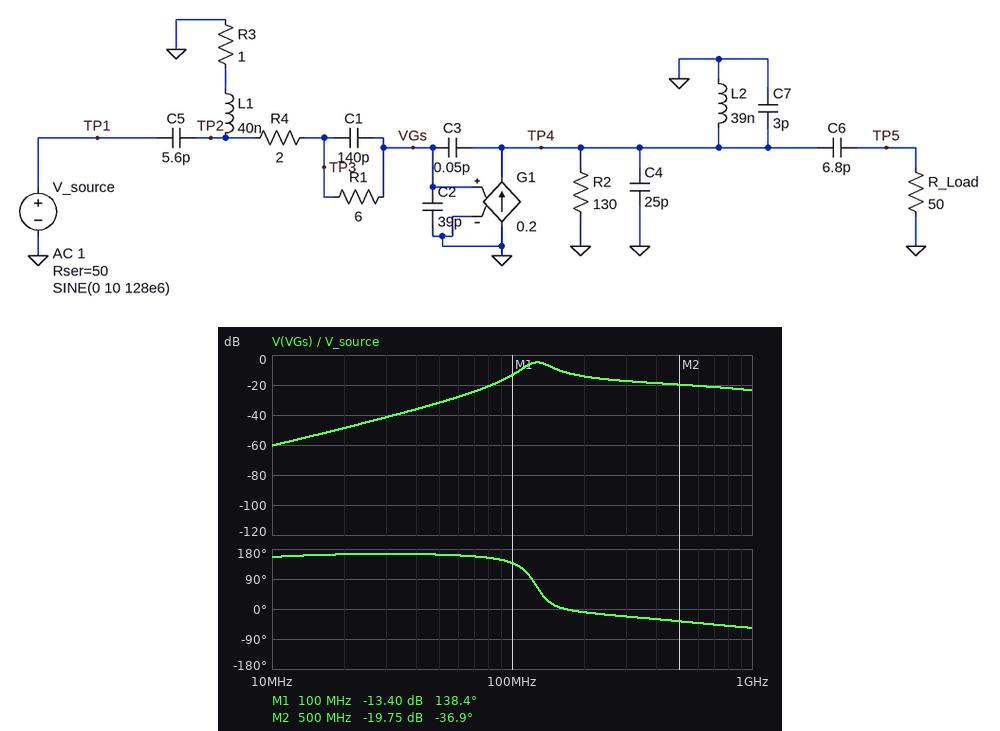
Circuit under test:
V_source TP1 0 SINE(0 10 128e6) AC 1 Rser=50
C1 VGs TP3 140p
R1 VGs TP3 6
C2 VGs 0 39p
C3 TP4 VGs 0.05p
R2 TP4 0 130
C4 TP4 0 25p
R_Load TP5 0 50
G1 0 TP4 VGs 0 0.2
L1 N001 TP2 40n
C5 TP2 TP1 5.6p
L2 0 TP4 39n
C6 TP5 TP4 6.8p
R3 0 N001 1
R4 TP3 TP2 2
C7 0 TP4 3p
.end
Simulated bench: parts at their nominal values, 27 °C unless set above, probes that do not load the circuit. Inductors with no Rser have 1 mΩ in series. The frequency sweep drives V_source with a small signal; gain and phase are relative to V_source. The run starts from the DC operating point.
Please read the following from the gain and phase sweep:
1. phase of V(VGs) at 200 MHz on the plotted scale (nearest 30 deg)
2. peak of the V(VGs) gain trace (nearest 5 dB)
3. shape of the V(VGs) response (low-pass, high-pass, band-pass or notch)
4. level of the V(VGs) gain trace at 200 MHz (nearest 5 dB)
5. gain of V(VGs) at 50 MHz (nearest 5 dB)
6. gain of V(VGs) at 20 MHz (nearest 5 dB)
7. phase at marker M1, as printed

0 deg
-5 dB
band-pass
-15 dB
-30 dB
-50 dB
138.4 deg
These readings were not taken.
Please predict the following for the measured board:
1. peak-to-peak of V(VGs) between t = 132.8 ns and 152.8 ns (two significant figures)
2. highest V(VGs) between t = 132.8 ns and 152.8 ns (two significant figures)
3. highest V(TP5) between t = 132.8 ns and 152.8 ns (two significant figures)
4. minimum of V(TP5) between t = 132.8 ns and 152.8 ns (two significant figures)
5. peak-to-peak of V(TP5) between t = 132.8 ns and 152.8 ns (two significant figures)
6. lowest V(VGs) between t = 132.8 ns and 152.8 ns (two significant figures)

11 V
5.7 V
30 V
-30 V
60 V
-5.7 V
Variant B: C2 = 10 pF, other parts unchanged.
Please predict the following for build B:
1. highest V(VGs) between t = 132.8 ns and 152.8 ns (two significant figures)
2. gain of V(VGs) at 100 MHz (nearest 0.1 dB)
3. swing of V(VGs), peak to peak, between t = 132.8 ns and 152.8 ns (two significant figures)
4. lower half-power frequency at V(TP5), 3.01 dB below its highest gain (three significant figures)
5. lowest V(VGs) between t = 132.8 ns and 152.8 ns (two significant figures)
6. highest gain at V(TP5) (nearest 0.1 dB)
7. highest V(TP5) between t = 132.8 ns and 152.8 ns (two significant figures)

2.2 V
-19.0 dB
4.3 V
189 MHz
-2.2 V
16.4 dB
11 V
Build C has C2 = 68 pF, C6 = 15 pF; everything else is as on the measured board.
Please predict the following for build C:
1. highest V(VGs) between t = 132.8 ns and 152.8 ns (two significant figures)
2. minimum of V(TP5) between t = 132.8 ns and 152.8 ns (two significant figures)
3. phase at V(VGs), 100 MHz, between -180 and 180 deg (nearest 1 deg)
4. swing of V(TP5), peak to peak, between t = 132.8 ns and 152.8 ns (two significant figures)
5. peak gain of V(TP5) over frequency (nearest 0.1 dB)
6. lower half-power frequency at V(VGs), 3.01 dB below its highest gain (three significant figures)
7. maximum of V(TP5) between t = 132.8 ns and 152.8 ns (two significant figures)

1.7 V
-13 V
67 deg
26 V
3.1 dB
86.8 MHz
13 V
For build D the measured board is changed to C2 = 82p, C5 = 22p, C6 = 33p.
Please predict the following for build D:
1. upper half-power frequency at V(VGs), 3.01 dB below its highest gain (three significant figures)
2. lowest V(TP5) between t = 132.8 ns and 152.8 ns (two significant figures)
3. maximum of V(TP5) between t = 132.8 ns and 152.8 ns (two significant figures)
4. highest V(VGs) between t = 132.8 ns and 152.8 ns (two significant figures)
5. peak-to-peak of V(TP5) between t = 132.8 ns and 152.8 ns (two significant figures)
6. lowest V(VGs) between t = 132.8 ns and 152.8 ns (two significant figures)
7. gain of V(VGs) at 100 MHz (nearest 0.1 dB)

108 MHz
-21 V
21 V
2.7 V
42 V
-2.7 V
-7.8 dB
